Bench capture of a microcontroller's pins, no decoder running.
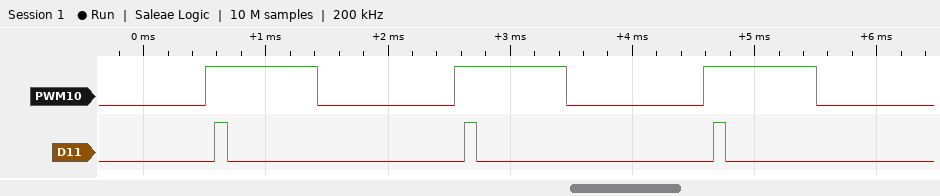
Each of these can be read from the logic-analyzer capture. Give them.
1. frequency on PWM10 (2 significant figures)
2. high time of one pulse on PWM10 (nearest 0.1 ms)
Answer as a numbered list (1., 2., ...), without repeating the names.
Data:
1. 490 Hz
2. 0.9 ms
